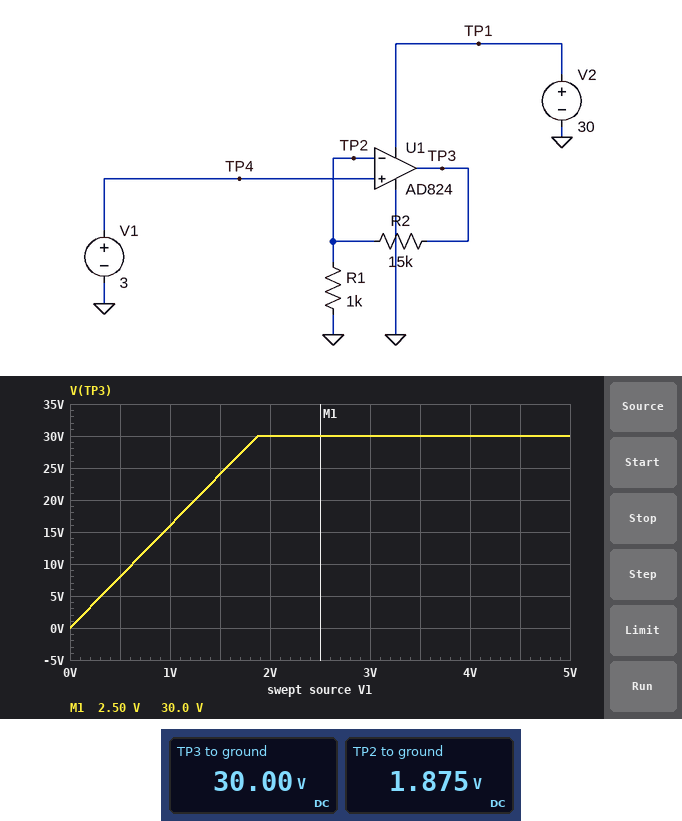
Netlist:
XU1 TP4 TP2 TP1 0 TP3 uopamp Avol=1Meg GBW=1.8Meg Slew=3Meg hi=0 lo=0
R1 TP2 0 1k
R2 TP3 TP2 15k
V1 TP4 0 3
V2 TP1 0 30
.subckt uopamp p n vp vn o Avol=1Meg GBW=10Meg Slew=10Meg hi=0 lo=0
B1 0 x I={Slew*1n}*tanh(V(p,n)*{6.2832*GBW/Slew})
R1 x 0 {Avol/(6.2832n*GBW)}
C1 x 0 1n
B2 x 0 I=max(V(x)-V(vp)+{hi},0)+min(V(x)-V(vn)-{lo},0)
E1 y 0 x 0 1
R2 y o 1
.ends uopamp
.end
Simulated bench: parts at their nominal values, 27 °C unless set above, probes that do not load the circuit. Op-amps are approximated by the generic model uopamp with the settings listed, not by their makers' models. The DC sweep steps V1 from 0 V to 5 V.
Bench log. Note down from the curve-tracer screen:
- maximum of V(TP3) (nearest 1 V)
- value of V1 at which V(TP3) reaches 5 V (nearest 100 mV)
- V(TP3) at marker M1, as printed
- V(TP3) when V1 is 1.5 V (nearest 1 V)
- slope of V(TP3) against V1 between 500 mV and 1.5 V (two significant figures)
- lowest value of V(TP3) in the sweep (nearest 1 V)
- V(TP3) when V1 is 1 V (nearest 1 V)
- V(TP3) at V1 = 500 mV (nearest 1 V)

30 V
300 mV
30.0 V
24 V
16 V/V
0 V
16 V
8 V
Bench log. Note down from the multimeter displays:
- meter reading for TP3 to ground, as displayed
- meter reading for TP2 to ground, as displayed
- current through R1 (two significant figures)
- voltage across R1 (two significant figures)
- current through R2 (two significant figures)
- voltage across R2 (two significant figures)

30.00 V
1.875 V
1.9 mA
1.9 V
1.9 mA
28 V
